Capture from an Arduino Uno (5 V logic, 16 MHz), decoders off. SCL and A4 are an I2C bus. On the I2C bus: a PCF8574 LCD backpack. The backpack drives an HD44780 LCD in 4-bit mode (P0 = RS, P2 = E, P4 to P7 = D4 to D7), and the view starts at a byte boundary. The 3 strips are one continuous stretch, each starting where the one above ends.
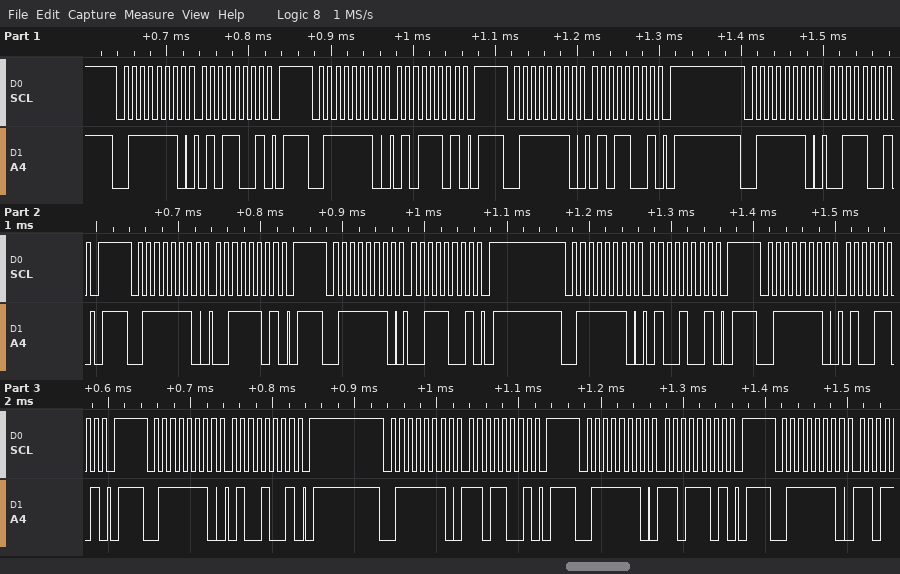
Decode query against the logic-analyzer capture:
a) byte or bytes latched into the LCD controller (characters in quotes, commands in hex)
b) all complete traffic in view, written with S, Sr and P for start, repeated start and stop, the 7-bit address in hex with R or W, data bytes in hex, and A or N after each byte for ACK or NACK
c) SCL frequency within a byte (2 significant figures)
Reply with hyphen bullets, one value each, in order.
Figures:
- 'S'
- S 3FW A 59 A P S 3FW A 5D A P S 3FW A 59 A P S 3FW A 39 A P S 3FW A 3D A P S 3FW A 39 A P S 3FW A 49 A P S 3FW A 4D A P S 3FW A 49 A P S 3FW A D9 A P S 3FW A DD A P S 3FW A
- 100 kHz
